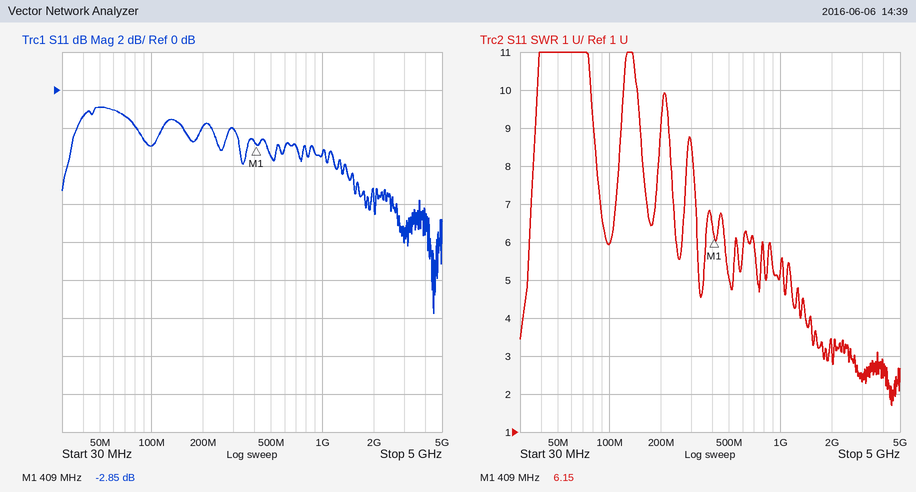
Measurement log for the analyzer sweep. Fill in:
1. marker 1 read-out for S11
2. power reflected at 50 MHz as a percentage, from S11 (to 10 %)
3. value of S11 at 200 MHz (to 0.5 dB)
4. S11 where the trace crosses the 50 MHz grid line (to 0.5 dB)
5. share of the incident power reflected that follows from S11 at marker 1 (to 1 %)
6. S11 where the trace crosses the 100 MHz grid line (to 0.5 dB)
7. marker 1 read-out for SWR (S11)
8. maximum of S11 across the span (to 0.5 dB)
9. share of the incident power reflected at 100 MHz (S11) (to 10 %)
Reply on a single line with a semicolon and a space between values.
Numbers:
-2.85 dB; 80 %; -2.0 dB; -1.0 dB; 52 %; -3.0 dB; 6.15; -1.0 dB; 50 %
